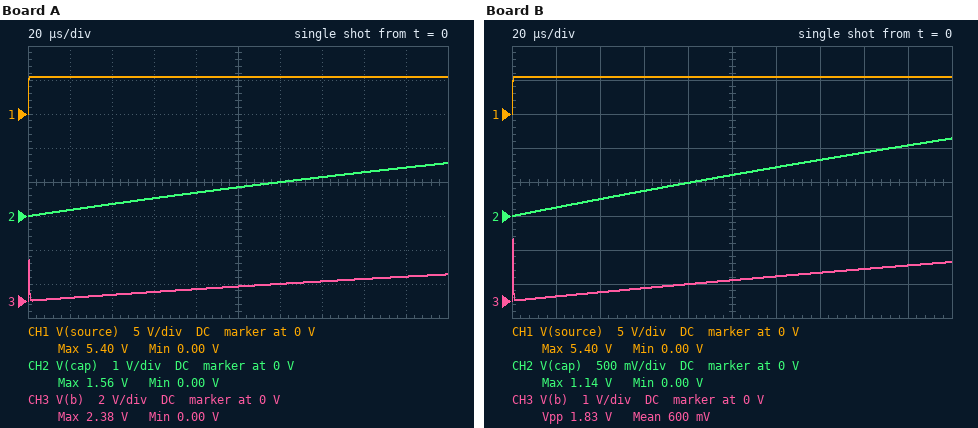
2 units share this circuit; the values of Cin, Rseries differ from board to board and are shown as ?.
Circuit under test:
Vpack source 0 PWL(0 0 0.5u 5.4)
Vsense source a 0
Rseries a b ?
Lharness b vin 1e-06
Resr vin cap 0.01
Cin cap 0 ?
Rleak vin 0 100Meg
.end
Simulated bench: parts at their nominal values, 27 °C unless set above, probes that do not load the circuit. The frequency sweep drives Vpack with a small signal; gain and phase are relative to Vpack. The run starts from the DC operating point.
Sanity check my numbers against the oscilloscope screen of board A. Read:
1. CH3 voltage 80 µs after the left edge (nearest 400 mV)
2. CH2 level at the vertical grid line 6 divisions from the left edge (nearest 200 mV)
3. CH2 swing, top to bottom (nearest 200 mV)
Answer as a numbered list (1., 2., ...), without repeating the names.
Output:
1. 800 mV
2. 1.0 V
3. 1.6 V
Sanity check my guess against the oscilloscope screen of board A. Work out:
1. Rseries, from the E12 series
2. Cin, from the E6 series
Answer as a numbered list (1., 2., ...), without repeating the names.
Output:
1. 3.9 Ω
2. 150 µF
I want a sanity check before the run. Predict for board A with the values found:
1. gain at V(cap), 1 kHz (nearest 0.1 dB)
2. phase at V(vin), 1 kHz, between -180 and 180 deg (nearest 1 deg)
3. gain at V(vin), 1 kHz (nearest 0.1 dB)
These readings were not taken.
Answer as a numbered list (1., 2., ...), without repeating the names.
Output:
1. -11.6 dB
2. -74 deg
3. -11.6 dB
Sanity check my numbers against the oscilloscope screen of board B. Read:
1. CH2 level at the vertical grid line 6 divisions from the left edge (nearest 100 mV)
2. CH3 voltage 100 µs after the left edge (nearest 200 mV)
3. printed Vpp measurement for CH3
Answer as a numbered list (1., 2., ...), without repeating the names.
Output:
1. 700 mV
2. 600 mV
3. 1.83 V
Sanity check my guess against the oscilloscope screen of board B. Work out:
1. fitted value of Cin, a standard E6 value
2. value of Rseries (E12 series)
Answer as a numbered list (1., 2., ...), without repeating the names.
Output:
1. 150 µF
2. 5.6 Ω
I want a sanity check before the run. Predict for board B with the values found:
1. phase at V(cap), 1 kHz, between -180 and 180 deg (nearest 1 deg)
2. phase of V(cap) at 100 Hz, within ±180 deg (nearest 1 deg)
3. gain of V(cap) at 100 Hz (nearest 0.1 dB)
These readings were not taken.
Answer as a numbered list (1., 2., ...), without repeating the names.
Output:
1. -79 deg
2. -28 deg
3. -1.1 dB
